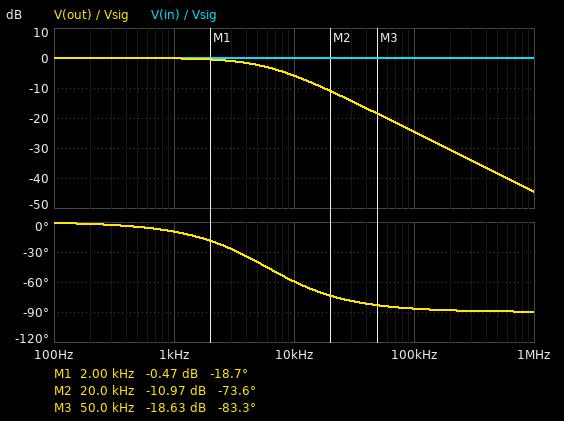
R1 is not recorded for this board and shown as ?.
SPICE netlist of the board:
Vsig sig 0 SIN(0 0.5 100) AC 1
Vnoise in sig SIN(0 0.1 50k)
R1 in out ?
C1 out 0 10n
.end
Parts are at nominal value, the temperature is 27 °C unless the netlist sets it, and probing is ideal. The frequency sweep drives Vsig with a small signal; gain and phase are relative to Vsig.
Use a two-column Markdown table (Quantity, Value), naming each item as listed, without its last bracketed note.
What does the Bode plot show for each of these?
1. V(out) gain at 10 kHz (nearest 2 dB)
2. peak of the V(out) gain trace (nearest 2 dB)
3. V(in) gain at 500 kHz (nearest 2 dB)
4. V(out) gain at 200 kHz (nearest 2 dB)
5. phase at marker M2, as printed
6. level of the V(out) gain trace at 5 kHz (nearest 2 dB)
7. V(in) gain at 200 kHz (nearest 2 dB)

| Quantity | Value |
|---|---|
| V(out) gain at 10 kHz | -6 dB |
| peak of the V(out) gain trace | 0 dB |
| V(in) gain at 500 kHz | 0 dB |
| V(out) gain at 200 kHz | -30 dB |
| phase at marker M2, as printed | -73.6 deg |
| level of the V(out) gain trace at 5 kHz | -2 dB |
| V(in) gain at 200 kHz | 0 dB |
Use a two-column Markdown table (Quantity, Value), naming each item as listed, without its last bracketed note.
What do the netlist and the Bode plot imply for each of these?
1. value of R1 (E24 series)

| Quantity | Value |
|---|---|
| value of R1 | 2.7 kΩ |
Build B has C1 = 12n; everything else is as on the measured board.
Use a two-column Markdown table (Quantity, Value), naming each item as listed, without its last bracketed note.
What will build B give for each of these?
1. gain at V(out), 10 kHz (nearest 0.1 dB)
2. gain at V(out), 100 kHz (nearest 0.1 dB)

| Quantity | Value |
|---|---|
| gain at V(out), 10 kHz | -7.1 dB |
| gain at V(out), 100 kHz | -26.2 dB |
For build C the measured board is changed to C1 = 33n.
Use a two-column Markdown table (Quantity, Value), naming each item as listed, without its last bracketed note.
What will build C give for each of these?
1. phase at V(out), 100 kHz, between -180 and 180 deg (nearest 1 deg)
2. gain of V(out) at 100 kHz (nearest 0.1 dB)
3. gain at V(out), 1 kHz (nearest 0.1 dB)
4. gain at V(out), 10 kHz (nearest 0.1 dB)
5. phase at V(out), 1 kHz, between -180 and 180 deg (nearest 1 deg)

| Quantity | Value |
|---|---|
| phase at V(out), 100 kHz, between -180 and 180 deg | -89 deg |
| gain of V(out) at 100 kHz | -35.0 dB |
| gain at V(out), 1 kHz | -1.2 dB |
| gain at V(out), 10 kHz | -15.1 dB |
| phase at V(out), 1 kHz, between -180 and 180 deg | -29 deg |
